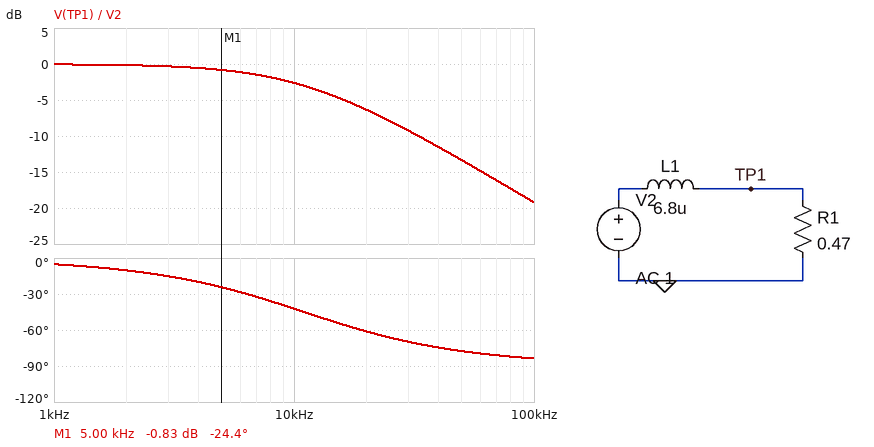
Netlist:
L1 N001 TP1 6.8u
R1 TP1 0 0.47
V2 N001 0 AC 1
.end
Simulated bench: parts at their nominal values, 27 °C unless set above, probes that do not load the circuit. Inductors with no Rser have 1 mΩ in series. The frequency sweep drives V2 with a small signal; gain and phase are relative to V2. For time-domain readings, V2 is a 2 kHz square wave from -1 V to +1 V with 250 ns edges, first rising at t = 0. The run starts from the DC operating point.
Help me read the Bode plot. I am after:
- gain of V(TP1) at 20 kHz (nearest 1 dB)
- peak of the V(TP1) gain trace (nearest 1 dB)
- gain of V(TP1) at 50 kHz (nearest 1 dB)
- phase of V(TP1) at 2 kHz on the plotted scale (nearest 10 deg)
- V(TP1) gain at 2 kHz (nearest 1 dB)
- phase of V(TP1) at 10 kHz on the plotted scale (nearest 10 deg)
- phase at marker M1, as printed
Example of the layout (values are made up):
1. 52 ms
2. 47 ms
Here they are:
1. -6 dB
2. 0 dB
3. -13 dB
4. -10 deg
5. 0 dB
6. -40 deg
7. -24.4 deg
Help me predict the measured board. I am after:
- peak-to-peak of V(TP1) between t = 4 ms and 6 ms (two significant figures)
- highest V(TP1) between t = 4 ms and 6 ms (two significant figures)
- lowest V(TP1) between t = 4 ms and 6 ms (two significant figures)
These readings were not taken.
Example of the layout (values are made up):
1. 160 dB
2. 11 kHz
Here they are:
1. 2.0 V
2. 1.0 V
3. -1.0 V
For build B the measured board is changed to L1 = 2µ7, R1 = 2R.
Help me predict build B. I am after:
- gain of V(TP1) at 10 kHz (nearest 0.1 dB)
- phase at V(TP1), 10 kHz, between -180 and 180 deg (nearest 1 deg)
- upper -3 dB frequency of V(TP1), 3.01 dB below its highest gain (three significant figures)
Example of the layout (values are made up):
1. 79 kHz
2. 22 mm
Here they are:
1. 0 dB
2. -5 deg
3. 118 kHz
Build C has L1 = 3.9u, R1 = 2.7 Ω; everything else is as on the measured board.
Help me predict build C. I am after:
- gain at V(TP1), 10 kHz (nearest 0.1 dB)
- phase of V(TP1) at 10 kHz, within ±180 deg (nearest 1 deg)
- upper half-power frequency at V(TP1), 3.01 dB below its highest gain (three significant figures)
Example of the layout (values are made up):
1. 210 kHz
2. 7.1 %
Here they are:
1. 0 dB
2. -5 deg
3. 110 kHz
